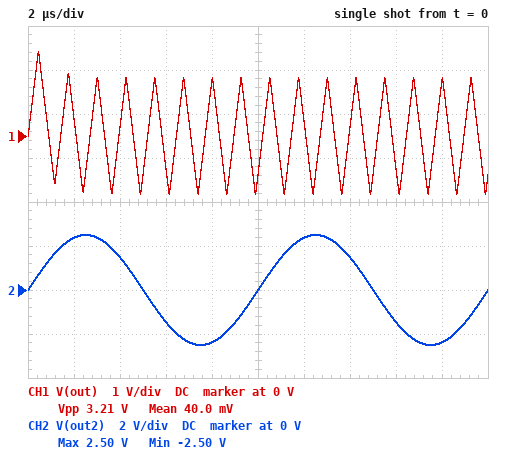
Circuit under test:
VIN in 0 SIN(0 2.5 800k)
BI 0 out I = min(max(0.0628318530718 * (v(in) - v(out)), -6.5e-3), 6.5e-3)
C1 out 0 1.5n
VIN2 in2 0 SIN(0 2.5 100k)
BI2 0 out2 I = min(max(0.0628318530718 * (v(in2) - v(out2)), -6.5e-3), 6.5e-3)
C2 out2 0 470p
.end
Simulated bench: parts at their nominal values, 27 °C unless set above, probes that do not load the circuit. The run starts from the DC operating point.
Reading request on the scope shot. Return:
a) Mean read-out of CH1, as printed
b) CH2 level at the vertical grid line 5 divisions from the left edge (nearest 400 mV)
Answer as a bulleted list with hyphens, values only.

- 40.0 mV
- 0 V
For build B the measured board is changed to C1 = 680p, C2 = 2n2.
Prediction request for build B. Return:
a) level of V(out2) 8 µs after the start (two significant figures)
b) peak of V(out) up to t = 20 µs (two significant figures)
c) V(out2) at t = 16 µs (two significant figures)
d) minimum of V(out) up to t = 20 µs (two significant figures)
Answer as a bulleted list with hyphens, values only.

- -2.4 V
- 2.5 V
- -1.4 V
- -2.5 V
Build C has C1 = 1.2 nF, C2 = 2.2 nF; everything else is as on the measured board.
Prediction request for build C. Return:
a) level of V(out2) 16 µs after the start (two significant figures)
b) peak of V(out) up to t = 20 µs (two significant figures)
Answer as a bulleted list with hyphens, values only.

- -1.4 V
- 2.2 V
